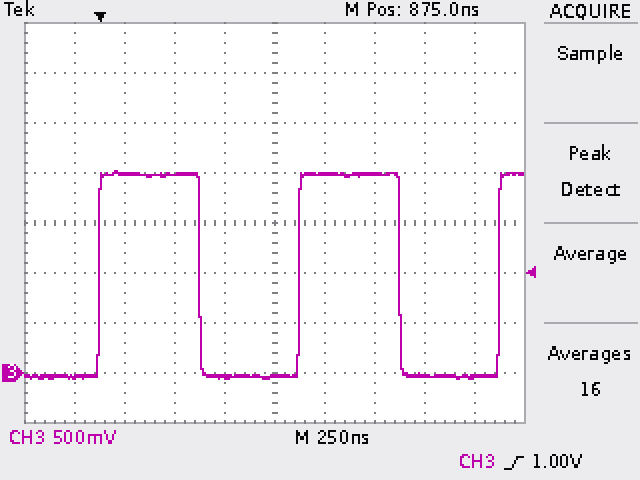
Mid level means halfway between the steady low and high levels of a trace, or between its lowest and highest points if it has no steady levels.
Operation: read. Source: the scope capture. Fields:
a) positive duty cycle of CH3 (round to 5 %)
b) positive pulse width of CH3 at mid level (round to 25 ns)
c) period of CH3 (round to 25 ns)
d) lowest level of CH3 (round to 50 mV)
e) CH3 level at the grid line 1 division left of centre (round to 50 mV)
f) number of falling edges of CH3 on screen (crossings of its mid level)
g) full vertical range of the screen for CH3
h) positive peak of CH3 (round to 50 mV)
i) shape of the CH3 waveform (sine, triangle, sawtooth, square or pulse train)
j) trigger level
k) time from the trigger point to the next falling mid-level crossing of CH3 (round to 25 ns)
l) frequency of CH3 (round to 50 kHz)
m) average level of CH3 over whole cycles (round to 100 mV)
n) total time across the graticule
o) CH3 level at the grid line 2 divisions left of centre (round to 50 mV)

50 %
500 ns
1.000 µs
-50 mV
-50 mV
2
4 V
2.00 V
square
1.00 V
500 ns
1.00 MHz
1.0 V
2.5 µs
2.00 V
